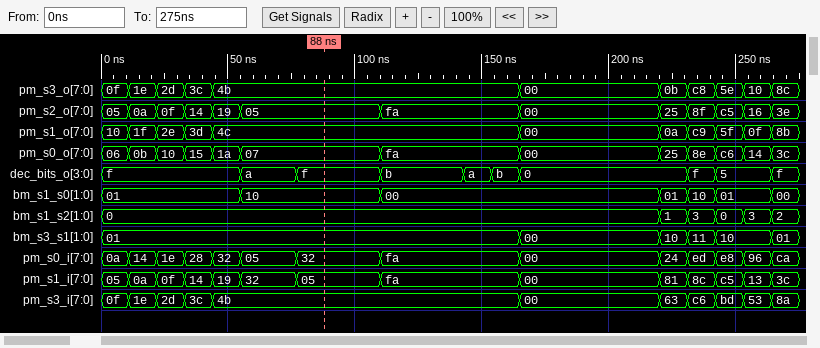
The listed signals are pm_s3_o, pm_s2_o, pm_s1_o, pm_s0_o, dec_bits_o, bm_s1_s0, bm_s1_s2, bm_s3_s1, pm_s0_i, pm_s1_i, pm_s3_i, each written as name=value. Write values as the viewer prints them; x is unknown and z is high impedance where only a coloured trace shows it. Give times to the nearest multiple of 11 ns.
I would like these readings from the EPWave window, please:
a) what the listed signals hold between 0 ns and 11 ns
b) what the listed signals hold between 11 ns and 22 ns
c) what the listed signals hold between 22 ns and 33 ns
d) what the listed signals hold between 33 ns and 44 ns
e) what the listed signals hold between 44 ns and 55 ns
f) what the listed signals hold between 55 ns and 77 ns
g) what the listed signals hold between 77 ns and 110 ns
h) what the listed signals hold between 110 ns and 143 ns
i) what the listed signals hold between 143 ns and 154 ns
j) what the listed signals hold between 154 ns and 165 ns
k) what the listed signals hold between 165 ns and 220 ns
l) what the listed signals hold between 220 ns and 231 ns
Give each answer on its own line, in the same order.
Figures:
pm_s3_o=0f, pm_s2_o=05, pm_s1_o=10, pm_s0_o=06, dec_bits_o=f, bm_s1_s0=01, bm_s1_s2=0, bm_s3_s1=01, pm_s0_i=0a, pm_s1_i=05, pm_s3_i=0f
pm_s3_o=1e, pm_s2_o=0a, pm_s1_o=1f, pm_s0_o=0b, dec_bits_o=f, bm_s1_s0=01, bm_s1_s2=0, bm_s3_s1=01, pm_s0_i=14, pm_s1_i=0a, pm_s3_i=1e
pm_s3_o=2d, pm_s2_o=0f, pm_s1_o=2e, pm_s0_o=10, dec_bits_o=f, bm_s1_s0=01, bm_s1_s2=0, bm_s3_s1=01, pm_s0_i=1e, pm_s1_i=0f, pm_s3_i=2d
pm_s3_o=3c, pm_s2_o=14, pm_s1_o=3d, pm_s0_o=15, dec_bits_o=f, bm_s1_s0=01, bm_s1_s2=0, bm_s3_s1=01, pm_s0_i=28, pm_s1_i=14, pm_s3_i=3c
pm_s3_o=4b, pm_s2_o=19, pm_s1_o=4c, pm_s0_o=1a, dec_bits_o=f, bm_s1_s0=01, bm_s1_s2=0, bm_s3_s1=01, pm_s0_i=32, pm_s1_i=19, pm_s3_i=4b
pm_s3_o=4b, pm_s2_o=05, pm_s1_o=4c, pm_s0_o=07, dec_bits_o=a, bm_s1_s0=10, bm_s1_s2=0, bm_s3_s1=01, pm_s0_i=05, pm_s1_i=32, pm_s3_i=4b
pm_s3_o=4b, pm_s2_o=05, pm_s1_o=4c, pm_s0_o=07, dec_bits_o=f, bm_s1_s0=10, bm_s1_s2=0, bm_s3_s1=01, pm_s0_i=32, pm_s1_i=05, pm_s3_i=4b
pm_s3_o=4b, pm_s2_o=fa, pm_s1_o=4c, pm_s0_o=fa, dec_bits_o=b, bm_s1_s0=00, bm_s1_s2=0, bm_s3_s1=01, pm_s0_i=fa, pm_s1_i=fa, pm_s3_i=4b
pm_s3_o=4b, pm_s2_o=fa, pm_s1_o=4c, pm_s0_o=fa, dec_bits_o=a, bm_s1_s0=00, bm_s1_s2=0, bm_s3_s1=01, pm_s0_i=fa, pm_s1_i=fa, pm_s3_i=4b
pm_s3_o=4b, pm_s2_o=fa, pm_s1_o=4c, pm_s0_o=fa, dec_bits_o=b, bm_s1_s0=00, bm_s1_s2=0, bm_s3_s1=01, pm_s0_i=fa, pm_s1_i=fa, pm_s3_i=4b
pm_s3_o=00, pm_s2_o=00, pm_s1_o=00, pm_s0_o=00, dec_bits_o=0, bm_s1_s0=00, bm_s1_s2=0, bm_s3_s1=00, pm_s0_i=00, pm_s1_i=00, pm_s3_i=00
pm_s3_o=0b, pm_s2_o=25, pm_s1_o=0a, pm_s0_o=25, dec_bits_o=0, bm_s1_s0=01, bm_s1_s2=1, bm_s3_s1=10, pm_s0_i=24, pm_s1_i=81, pm_s3_i=63
